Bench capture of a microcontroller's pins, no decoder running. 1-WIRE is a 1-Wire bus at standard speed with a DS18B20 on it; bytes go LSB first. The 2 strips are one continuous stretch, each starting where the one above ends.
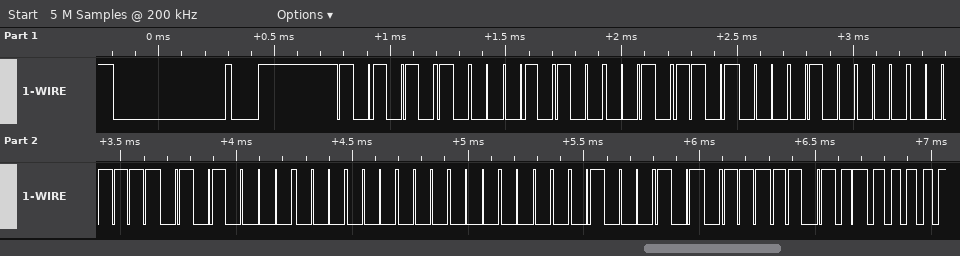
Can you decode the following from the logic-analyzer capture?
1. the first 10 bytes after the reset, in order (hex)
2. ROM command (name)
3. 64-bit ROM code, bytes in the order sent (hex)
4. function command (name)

55 28 B4 10 F0 0A 00 00 A2 BE
Match ROM
28 B4 10 F0 0A 00 00 A2
Read Scratchpad
